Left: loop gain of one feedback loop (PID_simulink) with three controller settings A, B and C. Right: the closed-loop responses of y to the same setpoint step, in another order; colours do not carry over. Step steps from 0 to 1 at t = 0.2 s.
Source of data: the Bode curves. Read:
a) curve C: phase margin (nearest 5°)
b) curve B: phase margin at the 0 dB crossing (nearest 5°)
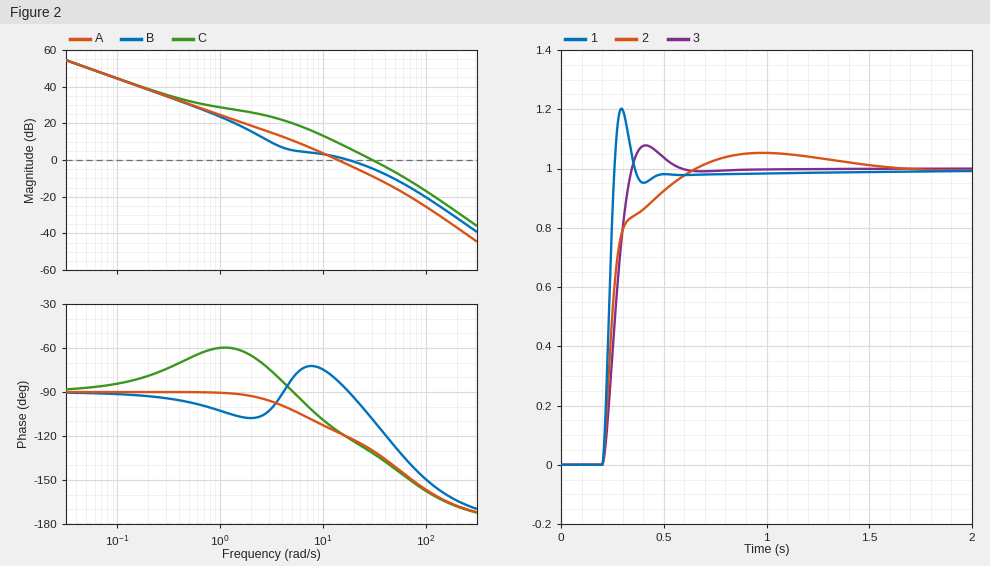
50°
90°
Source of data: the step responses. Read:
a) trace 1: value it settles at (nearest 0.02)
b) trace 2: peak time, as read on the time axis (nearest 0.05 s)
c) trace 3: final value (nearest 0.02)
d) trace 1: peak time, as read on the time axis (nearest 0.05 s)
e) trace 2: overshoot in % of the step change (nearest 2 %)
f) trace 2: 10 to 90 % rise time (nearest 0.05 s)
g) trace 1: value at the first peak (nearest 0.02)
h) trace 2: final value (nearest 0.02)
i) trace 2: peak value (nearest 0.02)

1.00
1.00 s
1.00
0.30 s
6 %
0.25 s
1.20
1.00
1.06
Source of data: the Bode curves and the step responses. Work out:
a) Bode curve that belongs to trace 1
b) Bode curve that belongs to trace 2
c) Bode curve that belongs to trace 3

C
B
A
